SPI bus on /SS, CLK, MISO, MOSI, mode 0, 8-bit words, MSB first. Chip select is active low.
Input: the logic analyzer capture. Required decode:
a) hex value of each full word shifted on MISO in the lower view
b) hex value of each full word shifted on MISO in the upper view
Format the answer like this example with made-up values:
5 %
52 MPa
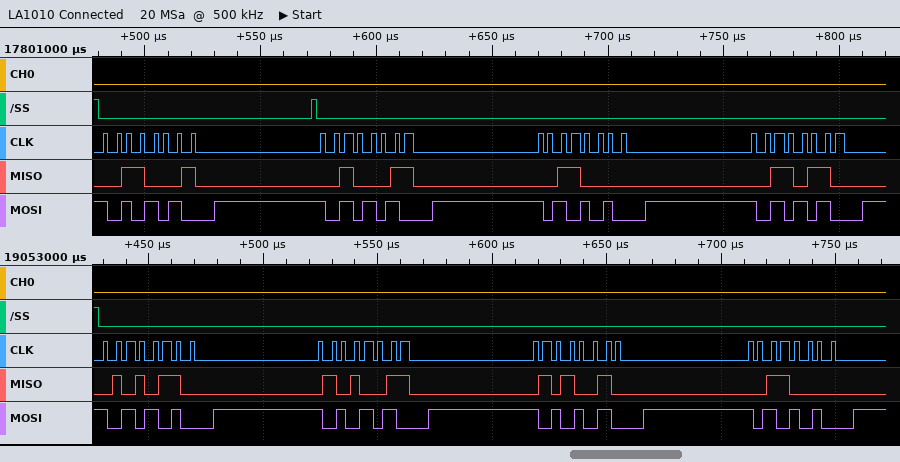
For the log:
56, 53, 52, 30
31, 23, 30, 36
